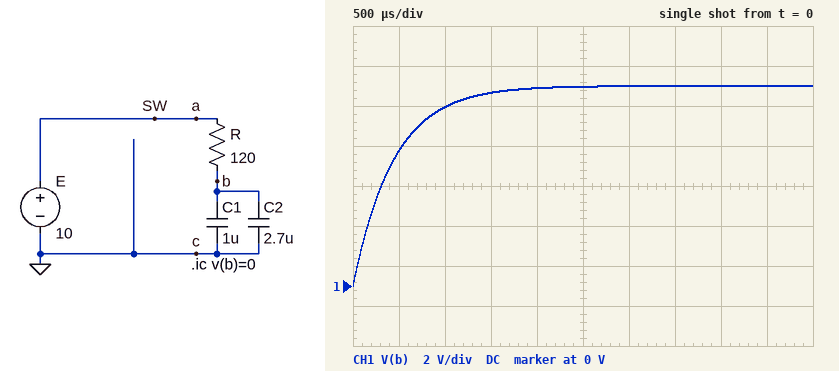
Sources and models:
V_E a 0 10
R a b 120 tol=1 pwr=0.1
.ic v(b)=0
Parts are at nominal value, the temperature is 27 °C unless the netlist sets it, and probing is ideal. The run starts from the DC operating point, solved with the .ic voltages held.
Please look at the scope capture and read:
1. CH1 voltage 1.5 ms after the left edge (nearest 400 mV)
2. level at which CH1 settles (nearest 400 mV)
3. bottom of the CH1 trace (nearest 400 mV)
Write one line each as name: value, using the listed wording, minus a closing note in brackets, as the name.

CH1 voltage 1.5 ms after the left edge: 9.6 V
level at which CH1 settles: 10.0 V
bottom of the CH1 trace: 0 V
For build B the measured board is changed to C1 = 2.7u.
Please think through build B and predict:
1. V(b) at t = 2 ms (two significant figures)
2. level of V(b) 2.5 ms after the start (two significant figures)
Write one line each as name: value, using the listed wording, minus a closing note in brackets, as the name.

V(b) at t = 2 ms: 9.5 V
level of V(b) 2.5 ms after the start: 9.8 V
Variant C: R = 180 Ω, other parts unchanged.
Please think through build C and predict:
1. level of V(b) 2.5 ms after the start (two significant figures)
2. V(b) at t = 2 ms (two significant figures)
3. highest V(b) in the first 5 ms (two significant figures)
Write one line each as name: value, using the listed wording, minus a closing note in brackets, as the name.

level of V(b) 2.5 ms after the start: 9.8 V
V(b) at t = 2 ms: 9.5 V
highest V(b) in the first 5 ms: 10 V
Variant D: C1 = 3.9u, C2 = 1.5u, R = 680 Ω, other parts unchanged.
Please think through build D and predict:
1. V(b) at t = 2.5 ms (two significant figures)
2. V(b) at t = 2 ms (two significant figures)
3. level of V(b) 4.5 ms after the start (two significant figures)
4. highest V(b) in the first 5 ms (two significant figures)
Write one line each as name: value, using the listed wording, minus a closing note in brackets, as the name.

V(b) at t = 2.5 ms: 4.9 V
V(b) at t = 2 ms: 4.2 V
level of V(b) 4.5 ms after the start: 7.1 V
highest V(b) in the first 5 ms: 7.4 V
